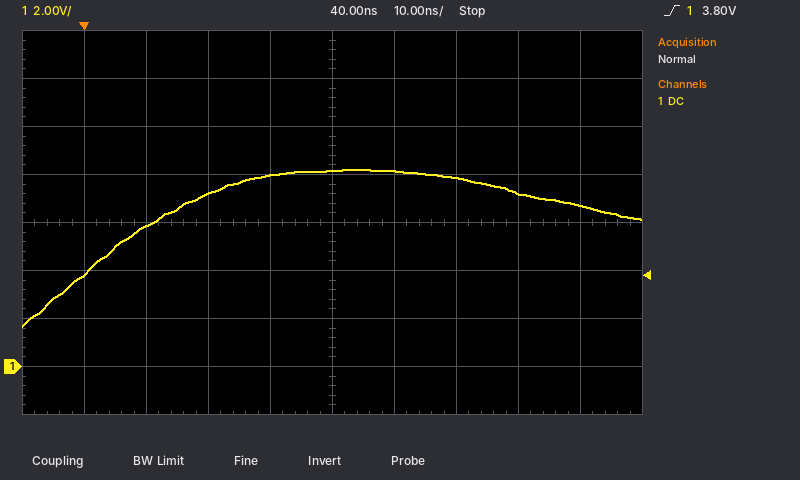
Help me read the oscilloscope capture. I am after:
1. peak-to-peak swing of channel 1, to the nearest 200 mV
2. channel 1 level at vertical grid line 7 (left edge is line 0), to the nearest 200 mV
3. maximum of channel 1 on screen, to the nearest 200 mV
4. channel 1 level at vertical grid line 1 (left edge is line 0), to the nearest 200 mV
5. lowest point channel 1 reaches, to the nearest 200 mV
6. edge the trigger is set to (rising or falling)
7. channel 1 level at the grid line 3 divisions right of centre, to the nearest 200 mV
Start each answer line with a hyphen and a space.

- 6.6 V
- 7.8 V
- 8.2 V
- 3.8 V
- 1.6 V
- rising
- 7.2 V
